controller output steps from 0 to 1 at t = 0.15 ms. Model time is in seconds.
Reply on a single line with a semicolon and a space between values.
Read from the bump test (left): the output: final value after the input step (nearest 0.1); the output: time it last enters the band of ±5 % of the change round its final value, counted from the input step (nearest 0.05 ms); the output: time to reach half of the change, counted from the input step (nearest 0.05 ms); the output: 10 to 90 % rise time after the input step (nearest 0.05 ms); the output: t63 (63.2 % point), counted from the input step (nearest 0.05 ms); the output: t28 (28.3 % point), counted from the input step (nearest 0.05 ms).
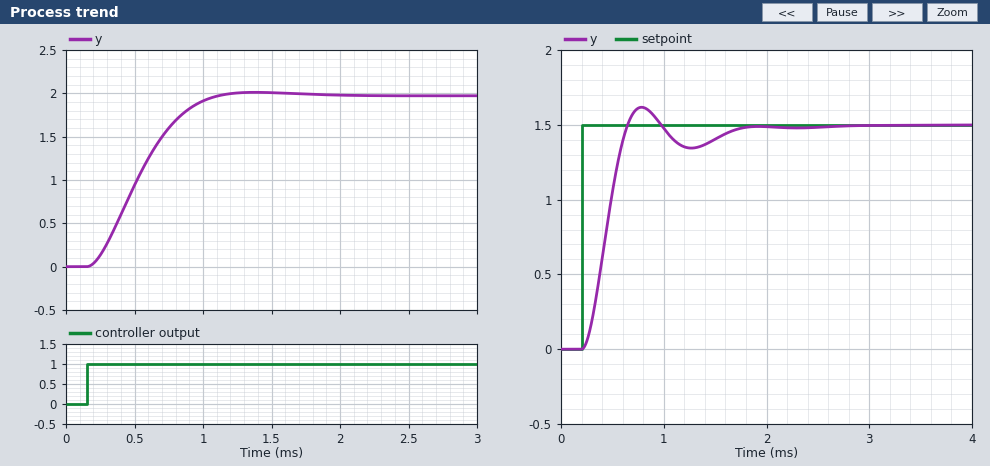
2.0; 0.80 ms; 0.35 ms; 0.60 ms; 0.45 ms; 0.25 ms
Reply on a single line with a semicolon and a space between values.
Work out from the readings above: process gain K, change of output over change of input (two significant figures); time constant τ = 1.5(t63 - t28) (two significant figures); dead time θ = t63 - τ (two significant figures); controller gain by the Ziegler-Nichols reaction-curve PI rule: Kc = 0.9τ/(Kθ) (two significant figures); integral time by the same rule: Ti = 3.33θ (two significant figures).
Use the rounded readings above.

2.0; 0.30 ms; 0.15 ms; 0.90; 0.50 ms
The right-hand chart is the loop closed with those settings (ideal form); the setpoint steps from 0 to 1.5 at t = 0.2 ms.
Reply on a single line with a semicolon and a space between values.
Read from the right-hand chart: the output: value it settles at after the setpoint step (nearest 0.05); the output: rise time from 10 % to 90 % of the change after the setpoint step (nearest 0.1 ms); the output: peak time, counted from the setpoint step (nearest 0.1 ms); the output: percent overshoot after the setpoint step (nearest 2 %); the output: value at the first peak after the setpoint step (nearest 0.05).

1.50; 0.3 ms; 0.6 ms; 8 %; 1.60
